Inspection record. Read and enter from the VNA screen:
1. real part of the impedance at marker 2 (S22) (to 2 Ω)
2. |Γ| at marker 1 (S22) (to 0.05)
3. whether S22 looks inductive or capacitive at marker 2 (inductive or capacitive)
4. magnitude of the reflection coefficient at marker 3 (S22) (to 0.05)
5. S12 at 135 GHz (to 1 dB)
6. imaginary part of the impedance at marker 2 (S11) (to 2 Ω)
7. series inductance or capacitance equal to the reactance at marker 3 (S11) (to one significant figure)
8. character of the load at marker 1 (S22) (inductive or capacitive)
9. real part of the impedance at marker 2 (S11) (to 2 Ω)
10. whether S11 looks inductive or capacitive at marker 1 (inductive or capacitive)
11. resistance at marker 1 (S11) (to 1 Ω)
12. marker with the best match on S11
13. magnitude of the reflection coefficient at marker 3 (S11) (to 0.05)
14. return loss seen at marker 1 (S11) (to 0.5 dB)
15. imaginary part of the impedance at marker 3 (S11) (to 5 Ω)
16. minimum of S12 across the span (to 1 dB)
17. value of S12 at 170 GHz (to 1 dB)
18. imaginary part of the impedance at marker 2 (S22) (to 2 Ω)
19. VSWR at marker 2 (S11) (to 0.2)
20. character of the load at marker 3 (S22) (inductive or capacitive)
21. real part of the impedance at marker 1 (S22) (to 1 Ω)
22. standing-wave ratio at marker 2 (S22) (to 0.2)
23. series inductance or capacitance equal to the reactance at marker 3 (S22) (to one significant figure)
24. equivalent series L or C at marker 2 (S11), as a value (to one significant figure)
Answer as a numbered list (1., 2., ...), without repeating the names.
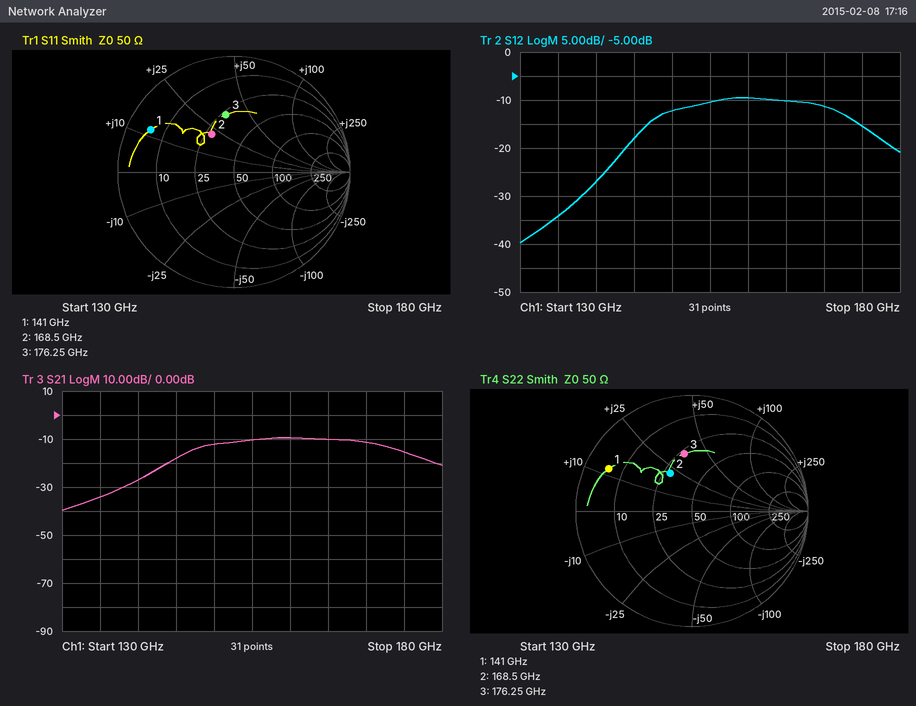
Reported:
1. 28 Ω
2. 0.80
3. inductive
4. 0.50
5. -34 dB
6. +22 Ω
7. 30 pH
8. inductive
9. 28 Ω
10. inductive
11. 6 Ω
12. marker 2
13. 0.50
14. 2.0 dB
15. +35 Ω
16. -40 dB
17. -11 dB
18. +22 Ω
19. 2.2
20. inductive
21. 6 Ω
22. 2.2
23. 30 pH
24. 20 pH
